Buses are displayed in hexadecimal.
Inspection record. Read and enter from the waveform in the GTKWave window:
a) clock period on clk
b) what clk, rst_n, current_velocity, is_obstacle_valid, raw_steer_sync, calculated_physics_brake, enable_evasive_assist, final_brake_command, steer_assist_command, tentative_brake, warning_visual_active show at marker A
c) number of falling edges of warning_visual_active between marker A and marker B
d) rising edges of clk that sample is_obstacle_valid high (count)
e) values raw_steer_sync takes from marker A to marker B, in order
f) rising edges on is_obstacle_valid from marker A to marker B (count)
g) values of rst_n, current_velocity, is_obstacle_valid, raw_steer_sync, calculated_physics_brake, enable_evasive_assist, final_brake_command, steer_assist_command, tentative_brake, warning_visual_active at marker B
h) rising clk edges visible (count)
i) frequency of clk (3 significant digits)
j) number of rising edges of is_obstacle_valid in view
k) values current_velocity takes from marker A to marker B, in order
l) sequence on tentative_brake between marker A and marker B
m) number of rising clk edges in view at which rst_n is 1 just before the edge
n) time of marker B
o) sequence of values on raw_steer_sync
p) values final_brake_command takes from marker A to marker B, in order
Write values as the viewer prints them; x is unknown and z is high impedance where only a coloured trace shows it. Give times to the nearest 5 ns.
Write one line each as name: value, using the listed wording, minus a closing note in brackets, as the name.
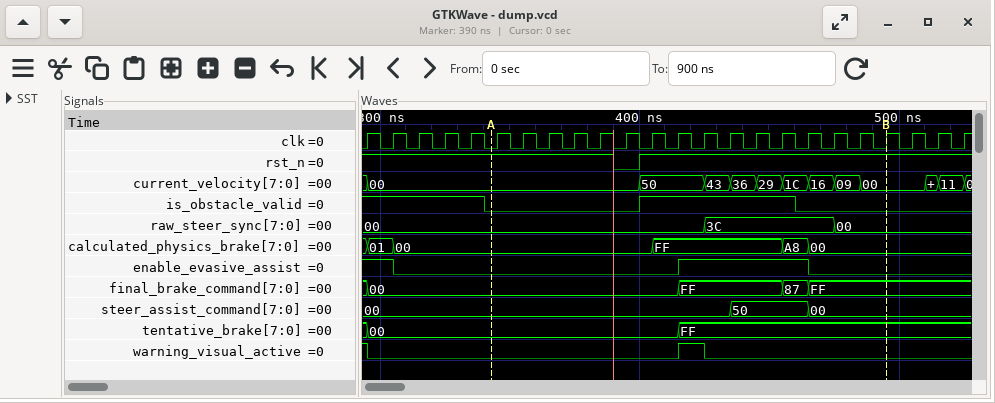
clock period on clk: 10 ns
what clk, rst_n, current_velocity, is_obstacle_valid, raw_steer_sync, calculated_physics_brake, enable_evasive_assist, final_brake_command, steer_assist_command, tentative_brake, warning_visual_active show at marker A: clk=0, rst_n=1, current_velocity=00, is_obstacle_valid=0, raw_steer_sync=00, calculated_physics_brake=00, enable_evasive_assist=0, final_brake_command=00, steer_assist_command=00, tentative_brake=00, warning_visual_active=0
number of falling edges of warning_visual_active between marker A and marker B: 1
rising edges of clk that sample is_obstacle_valid high: 11
values raw_steer_sync takes from marker A to marker B, in order: 00, 3C, 00
rising edges on is_obstacle_valid from marker A to marker B: 1
values of rst_n, current_velocity, is_obstacle_valid, raw_steer_sync, calculated_physics_brake, enable_evasive_assist, final_brake_command, steer_assist_command, tentative_brake, warning_visual_active at marker B: rst_n=1, current_velocity=00, is_obstacle_valid=0, raw_steer_sync=00, calculated_physics_brake=00, enable_evasive_assist=0, final_brake_command=FF, steer_assist_command=00, tentative_brake=FF, warning_visual_active=0
rising clk edges visible: 24
frequency of clk: 100 MHz
number of rising edges of is_obstacle_valid in view: 1
values current_velocity takes from marker A to marker B, in order: 00, 50, 43, 36, 29, 1C, 16, 09, 00
sequence on tentative_brake between marker A and marker B: 00, FF
number of rising clk edges in view at which rst_n is 1 just before the edge: 23
time of marker B: 495 ns
sequence of values on raw_steer_sync: 00, 3C, 00
values final_brake_command takes from marker A to marker B, in order: 00, FF, 87, FF
